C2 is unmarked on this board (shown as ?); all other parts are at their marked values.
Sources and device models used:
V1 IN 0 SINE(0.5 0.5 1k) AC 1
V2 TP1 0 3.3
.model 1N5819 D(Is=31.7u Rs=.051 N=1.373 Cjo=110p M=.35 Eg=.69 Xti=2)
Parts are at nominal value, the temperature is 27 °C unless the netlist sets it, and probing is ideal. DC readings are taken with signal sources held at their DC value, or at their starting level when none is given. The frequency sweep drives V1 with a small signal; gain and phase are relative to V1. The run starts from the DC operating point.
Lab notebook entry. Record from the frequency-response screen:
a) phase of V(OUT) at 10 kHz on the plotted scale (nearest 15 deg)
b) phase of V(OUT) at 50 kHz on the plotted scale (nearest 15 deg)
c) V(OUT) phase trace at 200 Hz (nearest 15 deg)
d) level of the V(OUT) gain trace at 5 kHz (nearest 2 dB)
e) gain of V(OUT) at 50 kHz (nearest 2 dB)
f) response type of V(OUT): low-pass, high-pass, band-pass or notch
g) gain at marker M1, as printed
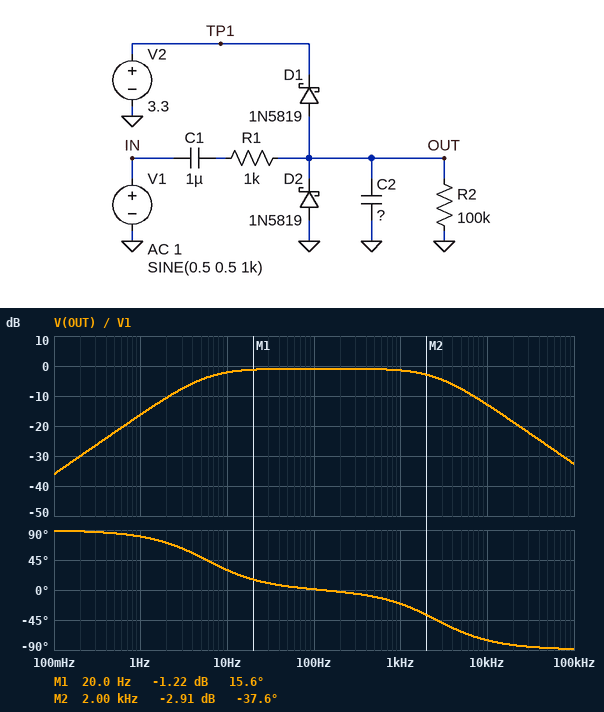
-75 deg
-90 deg
0 deg
-8 dB
-26 dB
band-pass
-1.22 dB
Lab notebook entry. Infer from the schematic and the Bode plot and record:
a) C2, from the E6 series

68 nF
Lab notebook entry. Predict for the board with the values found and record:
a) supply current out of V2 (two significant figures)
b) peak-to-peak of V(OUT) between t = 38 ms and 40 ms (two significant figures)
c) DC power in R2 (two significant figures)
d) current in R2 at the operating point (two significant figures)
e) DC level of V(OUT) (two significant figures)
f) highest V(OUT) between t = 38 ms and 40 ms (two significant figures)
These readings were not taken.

32 µA
840 mV
140 nW
1.2 µA
120 mV
840 mV
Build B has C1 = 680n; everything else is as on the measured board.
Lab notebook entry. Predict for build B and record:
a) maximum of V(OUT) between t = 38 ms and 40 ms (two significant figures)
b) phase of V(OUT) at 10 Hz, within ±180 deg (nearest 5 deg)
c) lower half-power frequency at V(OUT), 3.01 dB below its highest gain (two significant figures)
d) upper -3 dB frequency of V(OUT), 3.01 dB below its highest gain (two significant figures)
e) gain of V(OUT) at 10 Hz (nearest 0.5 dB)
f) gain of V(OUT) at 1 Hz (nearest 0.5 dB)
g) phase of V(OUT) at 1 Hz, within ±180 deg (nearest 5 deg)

820 mV
40 deg
8.2 Hz
2.7 kHz
-3.5 dB
-19.5 dB
85 deg
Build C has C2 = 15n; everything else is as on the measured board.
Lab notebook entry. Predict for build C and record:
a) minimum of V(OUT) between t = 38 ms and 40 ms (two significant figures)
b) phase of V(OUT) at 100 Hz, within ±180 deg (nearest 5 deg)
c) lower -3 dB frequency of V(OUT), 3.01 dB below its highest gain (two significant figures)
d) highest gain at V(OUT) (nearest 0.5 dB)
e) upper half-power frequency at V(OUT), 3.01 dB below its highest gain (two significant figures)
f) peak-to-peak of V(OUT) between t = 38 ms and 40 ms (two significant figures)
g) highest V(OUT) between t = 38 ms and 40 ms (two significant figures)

-4.9 mV
5 deg
6.0 Hz
-0.5 dB
11 kHz
940 mV
930 mV
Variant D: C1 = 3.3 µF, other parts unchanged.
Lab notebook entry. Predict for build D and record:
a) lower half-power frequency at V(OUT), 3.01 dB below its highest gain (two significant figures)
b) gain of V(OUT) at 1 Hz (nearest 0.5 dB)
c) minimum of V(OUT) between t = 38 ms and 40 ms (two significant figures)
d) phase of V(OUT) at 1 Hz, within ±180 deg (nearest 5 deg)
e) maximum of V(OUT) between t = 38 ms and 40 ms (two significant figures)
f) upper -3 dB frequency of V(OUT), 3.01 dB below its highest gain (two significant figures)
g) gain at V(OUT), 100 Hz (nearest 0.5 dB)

1.8 Hz
-7.0 dB
-29 mV
60 deg
820 mV
2.5 kHz
-0.5 dB
